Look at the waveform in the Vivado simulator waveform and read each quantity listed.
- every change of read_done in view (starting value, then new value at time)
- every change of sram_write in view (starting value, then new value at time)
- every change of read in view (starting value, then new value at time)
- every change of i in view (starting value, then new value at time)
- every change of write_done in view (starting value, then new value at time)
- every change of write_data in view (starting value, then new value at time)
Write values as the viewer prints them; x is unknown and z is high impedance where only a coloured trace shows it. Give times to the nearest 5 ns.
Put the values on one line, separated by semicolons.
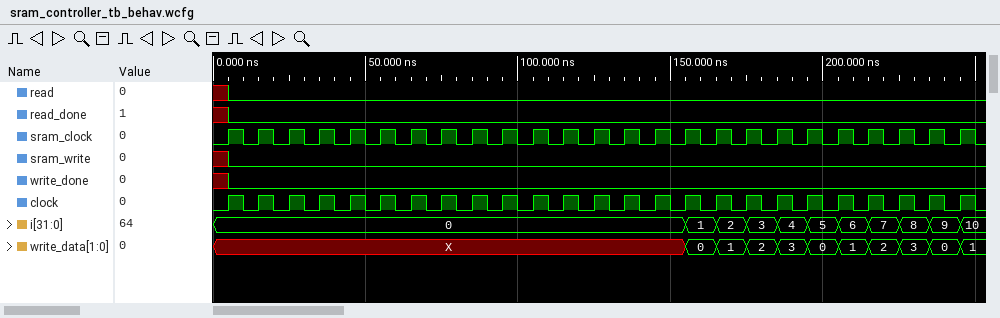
x, 0 at 5 ns; x, 0 at 5 ns; x, 0 at 5 ns; 0, 1 at 155 ns, 2 at 165 ns, 3 at 175 ns, 4 at 185 ns, 5 at 195 ns, 6 at 205 ns, 7 at 215 ns, 8 at 225 ns, 9 at 235 ns, 10 at 245 ns; x, 0 at 5 ns; X, 0 at 155 ns, 1 at 165 ns, 2 at 175 ns, 3 at 185 ns, 0 at 195 ns, 1 at 205 ns, 2 at 215 ns, 3 at 225 ns, 0 at 235 ns, 1 at 245 ns
